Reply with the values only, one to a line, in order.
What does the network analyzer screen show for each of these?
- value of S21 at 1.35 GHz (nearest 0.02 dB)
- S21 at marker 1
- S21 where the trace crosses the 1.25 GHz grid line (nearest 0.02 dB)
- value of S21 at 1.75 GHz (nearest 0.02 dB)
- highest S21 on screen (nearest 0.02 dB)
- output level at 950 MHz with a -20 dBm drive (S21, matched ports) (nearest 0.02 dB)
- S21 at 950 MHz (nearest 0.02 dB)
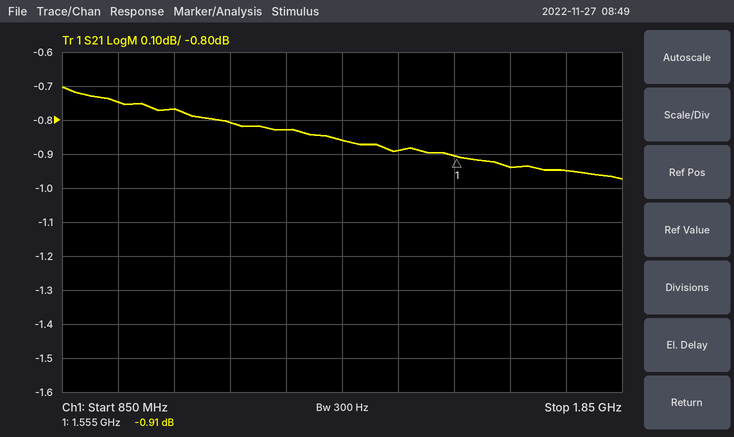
-0.86 dB
-0.91 dB
-0.82 dB
-0.94 dB
-0.70 dB
-20.74 dBm
-0.74 dB
